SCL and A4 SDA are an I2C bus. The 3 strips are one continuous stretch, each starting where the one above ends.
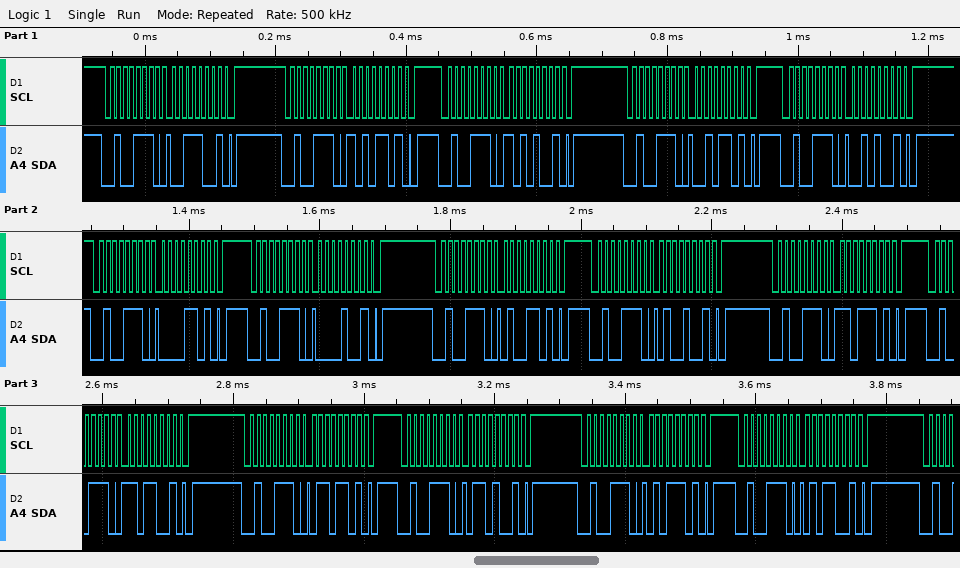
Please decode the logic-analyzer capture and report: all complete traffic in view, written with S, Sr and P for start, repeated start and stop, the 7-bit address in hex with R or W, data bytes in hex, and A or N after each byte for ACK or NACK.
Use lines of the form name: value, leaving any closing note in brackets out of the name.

all complete traffic in view, written with S, Sr and P for start, repeated start and stop, the 7-bit address in hex with R or W, data bytes in hex, and A or N after each byte for ACK or NACK: S 27W A 39 A P S 27W A AD A P S 27W A A9 A P S 27W A 2D A P S 27W A 29 A P S 27W A 0D A P S 27W A 09 A P S 27W A 4D A P S 27W A 49 A P S 27W A DD A P S 27W A D9 A P S 27W A 6D A P S 27W A 69 A P S 27W A 5D A P S 27W A 59 A P
